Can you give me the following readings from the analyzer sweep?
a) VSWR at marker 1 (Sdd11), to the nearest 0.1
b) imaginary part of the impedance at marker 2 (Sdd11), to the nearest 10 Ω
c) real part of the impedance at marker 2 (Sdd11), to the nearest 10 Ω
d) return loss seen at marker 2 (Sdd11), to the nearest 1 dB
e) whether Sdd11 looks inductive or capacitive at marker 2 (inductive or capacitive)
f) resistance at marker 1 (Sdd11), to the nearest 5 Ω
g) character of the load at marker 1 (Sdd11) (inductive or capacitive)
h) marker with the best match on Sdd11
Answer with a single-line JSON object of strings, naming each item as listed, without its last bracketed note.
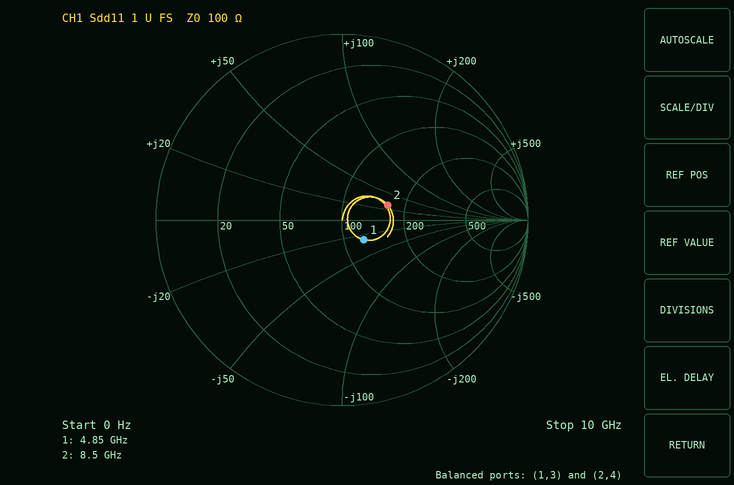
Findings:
{"VSWR at marker 1 (Sdd11), to the nearest 0.1": "1.4", "imaginary part of the impedance at marker 2 (Sdd11), to the nearest 10 Ω": "+30 Ω", "real part of the impedance at marker 2 (Sdd11), to the nearest 10 Ω": "160 Ω", "return loss seen at marker 2 (Sdd11), to the nearest 1 dB": "12 dB", "whether Sdd11 looks inductive or capacitive at marker 2": "inductive", "resistance at marker 1 (Sdd11), to the nearest 5 Ω": "125 Ω", "character of the load at marker 1 (Sdd11)": "capacitive", "marker with the best match on Sdd11": "marker 1"}
